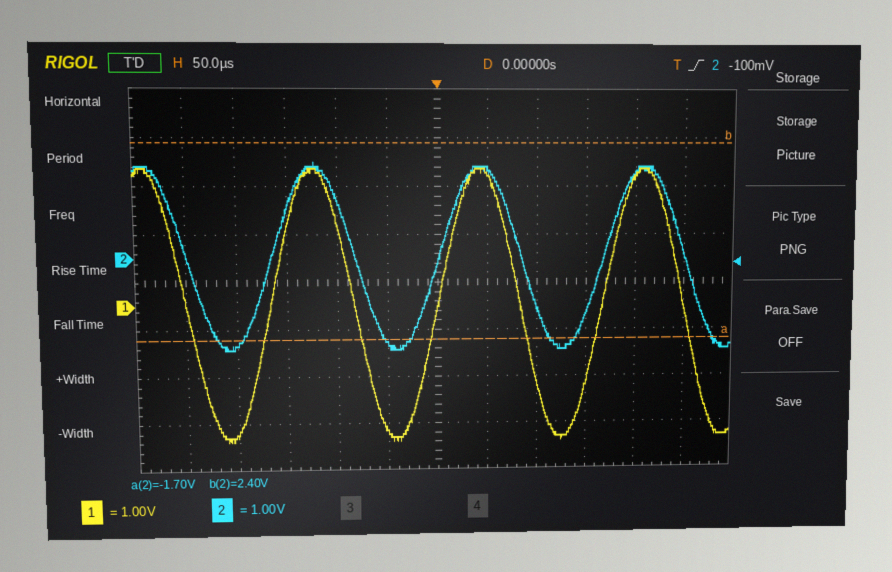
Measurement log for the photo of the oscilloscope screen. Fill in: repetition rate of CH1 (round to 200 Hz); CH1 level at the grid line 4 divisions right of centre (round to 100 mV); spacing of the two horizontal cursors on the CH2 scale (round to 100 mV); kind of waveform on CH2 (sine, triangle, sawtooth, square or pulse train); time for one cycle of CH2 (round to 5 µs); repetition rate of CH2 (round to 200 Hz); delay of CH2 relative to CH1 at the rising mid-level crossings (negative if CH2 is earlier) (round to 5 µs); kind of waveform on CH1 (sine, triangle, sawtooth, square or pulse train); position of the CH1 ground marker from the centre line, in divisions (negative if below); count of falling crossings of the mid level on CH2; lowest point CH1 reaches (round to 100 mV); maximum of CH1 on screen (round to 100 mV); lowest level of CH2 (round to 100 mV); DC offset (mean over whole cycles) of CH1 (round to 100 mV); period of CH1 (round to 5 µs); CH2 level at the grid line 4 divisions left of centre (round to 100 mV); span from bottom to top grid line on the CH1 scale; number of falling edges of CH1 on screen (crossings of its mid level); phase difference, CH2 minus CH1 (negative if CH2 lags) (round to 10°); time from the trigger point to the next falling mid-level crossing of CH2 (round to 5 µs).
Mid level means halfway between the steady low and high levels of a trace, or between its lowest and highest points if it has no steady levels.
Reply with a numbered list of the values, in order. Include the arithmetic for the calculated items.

1. 1 / 165 µs ≈ 6.06 kHz, so 6.0 kHz to the nearest 200 Hz
2. 2.7 V
3. 4.1 V
4. sine
5. 165 µs
6. 1 / 165 µs ≈ 6.06 kHz, so 6.0 kHz to the nearest 200 Hz
7. 0 µs
8. sine
9. -0.5 div
10. 4
11. -2.9 V
12. 2.9 V
13. -1.9 V
14. (2.9 V + (-2.9 V)) / 2 ≈ 0.0 V
15. 165 µs
16. -1.8 V
17. 8 V
18. 4
19. −360° × (0 µs) / 165 µs ≈ 0°
20. 85 µs
